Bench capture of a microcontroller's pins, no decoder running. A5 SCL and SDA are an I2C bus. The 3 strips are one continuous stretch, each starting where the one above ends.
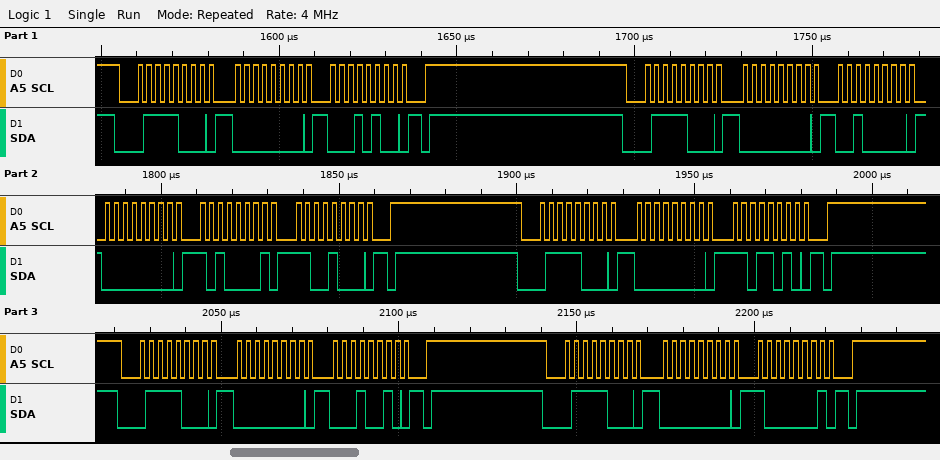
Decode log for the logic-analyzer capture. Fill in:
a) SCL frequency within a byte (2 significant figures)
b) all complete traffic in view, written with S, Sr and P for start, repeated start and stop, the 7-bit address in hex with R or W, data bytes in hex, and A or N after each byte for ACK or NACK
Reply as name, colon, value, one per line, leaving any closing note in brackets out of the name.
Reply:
SCL frequency within a byte: 400 kHz
all complete traffic in view, written with S, Sr and P for start, repeated start and stop, the 7-bit address in hex with R or W, data bytes in hex, and A or N after each byte for ACK or NACK: S 3CW A 00 A 14 A P S 3CW A 00 A 20 A 00 A A1 A C8 A P S 3CW A 00 A DA A P S 3CW A 00 A 12 A P S 3CW A 00 A 81 A P
